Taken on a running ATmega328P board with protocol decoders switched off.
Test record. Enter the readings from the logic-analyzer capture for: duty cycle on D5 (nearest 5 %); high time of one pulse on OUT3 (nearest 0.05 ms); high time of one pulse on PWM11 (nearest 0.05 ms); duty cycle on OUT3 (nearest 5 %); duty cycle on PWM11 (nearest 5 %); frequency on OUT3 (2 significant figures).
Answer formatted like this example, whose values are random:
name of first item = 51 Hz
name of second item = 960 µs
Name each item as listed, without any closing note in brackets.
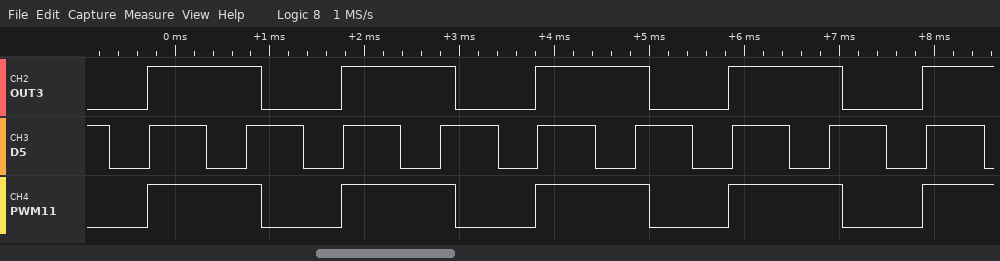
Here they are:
duty cycle on D5 = 60 %
high time of one pulse on OUT3 = 1.20 ms
high time of one pulse on PWM11 = 1.20 ms
duty cycle on OUT3 = 60 %
duty cycle on PWM11 = 60 %
frequency on OUT3 = 490 Hz
